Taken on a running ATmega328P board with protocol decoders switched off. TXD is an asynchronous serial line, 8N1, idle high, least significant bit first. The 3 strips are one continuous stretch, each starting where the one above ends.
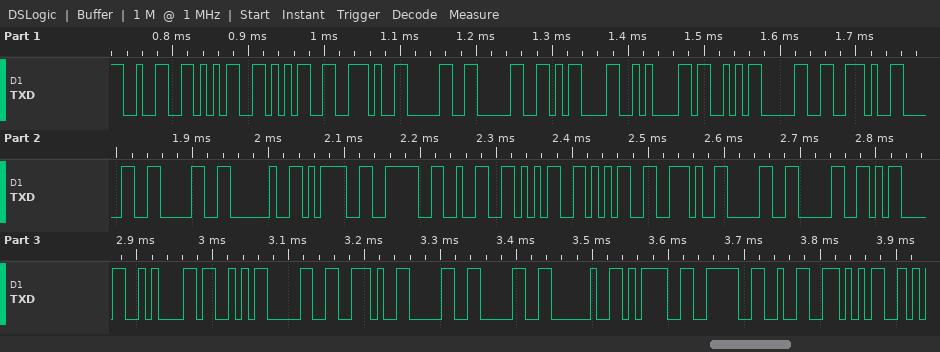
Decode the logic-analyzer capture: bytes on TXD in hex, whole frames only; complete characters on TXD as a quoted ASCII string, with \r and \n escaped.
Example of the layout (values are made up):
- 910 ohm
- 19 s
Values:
- 32 35 35 2E 30 30 0D 0A 53 30 2E 30 30 20 3D 3E 32 35 35 2E 30 30 0D 0A 53 30 2E 30 30 20 3D 3E 32 35
- "255.00\r\nS0.00 =>255.00\r\nS0.00 =>25"
